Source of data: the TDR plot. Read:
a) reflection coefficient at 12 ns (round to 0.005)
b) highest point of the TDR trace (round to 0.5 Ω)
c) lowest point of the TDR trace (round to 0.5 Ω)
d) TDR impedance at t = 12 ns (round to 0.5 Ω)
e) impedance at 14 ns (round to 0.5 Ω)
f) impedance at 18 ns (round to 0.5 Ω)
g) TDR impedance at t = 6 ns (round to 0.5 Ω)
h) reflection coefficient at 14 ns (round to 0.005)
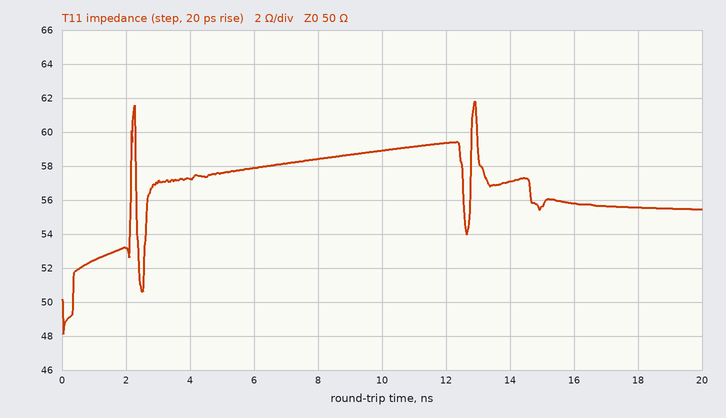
+0.085
62.0 Ω
48.0 Ω
59.5 Ω
57.0 Ω
55.5 Ω
58.0 Ω
+0.065
